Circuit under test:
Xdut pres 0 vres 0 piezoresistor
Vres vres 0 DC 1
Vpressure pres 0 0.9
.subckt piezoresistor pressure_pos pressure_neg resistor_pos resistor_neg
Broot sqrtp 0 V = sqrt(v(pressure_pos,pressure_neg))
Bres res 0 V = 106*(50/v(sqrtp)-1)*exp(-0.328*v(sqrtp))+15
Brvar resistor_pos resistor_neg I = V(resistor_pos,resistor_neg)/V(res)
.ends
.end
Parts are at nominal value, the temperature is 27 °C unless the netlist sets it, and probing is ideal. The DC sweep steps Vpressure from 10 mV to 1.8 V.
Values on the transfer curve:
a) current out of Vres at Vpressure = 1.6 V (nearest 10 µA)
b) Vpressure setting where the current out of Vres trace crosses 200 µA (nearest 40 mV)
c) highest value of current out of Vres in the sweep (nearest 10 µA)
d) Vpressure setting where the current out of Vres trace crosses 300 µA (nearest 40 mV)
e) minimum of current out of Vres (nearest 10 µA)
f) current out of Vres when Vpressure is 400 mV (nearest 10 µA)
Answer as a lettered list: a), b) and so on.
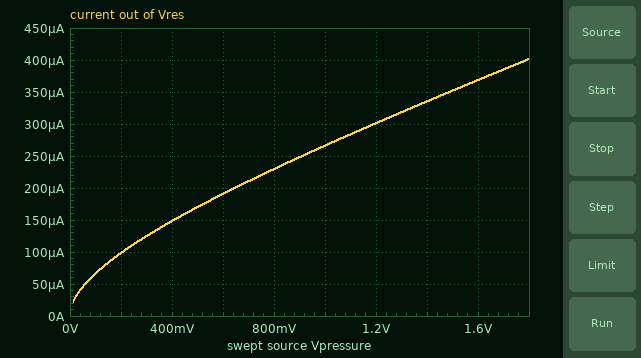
a) 370 µA
b) 640 mV
c) 400 µA
d) 1.20 V
e) 20 µA
f) 150 µA
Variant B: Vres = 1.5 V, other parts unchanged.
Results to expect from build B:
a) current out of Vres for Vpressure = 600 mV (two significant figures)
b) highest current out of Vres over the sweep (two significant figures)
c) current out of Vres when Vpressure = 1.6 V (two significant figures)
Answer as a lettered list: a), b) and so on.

a) 290 µA
b) 600 µA
c) 550 µA
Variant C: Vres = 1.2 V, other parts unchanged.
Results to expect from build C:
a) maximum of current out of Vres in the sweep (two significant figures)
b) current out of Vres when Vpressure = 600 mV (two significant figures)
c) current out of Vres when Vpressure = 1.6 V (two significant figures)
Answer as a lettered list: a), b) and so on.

a) 480 µA
b) 230 µA
c) 440 µA
